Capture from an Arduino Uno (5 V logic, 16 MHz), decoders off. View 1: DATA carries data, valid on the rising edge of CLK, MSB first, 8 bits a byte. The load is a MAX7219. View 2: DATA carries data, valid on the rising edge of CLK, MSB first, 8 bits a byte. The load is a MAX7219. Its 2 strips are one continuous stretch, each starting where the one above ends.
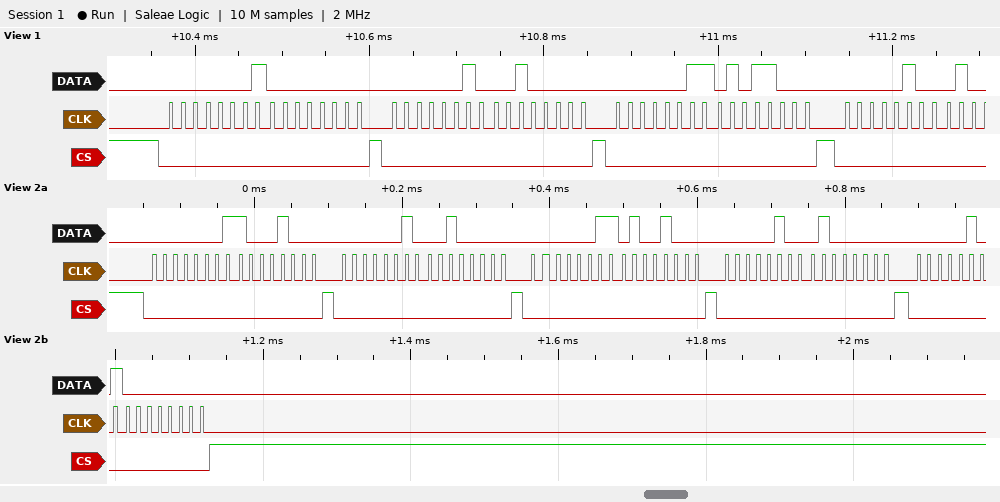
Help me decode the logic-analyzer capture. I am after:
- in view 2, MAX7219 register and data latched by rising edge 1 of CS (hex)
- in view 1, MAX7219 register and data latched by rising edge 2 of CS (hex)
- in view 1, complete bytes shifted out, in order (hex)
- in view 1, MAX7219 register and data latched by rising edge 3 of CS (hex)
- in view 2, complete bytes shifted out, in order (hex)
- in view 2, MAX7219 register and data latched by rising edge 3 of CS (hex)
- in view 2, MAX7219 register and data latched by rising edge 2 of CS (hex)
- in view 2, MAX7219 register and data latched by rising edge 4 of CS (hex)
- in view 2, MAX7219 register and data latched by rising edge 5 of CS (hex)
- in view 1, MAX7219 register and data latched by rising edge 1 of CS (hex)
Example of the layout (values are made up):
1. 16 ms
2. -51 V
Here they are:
1. register 0x1, data 0x88
2. register 0x2, data 0x20
3. 01 00 02 20 03 58 04
4. register 0x3, data 0x58
5. 01 88 02 20 03 48 04 40 05 00
6. register 0x3, data 0x48
7. register 0x2, data 0x20
8. register 0x4, data 0x40
9. register 0x5, data 0x00
10. register 0x1, data 0x00
